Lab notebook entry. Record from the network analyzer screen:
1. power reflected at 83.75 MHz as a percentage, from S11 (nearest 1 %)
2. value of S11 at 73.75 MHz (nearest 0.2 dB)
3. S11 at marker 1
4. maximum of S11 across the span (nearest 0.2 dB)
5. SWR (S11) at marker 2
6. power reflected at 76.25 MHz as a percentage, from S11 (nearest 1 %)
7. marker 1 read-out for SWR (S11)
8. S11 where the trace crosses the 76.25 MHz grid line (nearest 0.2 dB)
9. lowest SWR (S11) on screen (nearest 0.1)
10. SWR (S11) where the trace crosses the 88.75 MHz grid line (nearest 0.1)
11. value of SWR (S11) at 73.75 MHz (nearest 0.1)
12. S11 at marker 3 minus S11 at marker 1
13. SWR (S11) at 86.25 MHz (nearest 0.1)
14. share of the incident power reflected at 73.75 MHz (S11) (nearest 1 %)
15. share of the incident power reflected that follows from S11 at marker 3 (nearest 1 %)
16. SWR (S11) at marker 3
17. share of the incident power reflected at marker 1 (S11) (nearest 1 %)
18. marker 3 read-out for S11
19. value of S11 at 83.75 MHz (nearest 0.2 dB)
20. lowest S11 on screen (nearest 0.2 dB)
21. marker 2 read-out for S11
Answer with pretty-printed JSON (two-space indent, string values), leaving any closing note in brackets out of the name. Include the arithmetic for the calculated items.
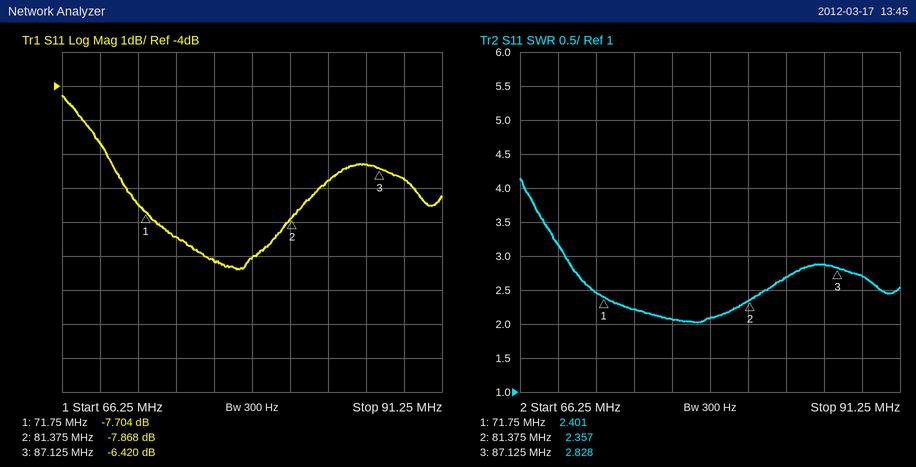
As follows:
{
  "power reflected at 83.75 MHz as a percentage, from S11": "10^(-6.8/10) ≈ 21 %",
  "value of S11 at 73.75 MHz": "-8.4 dB",
  "S11 at marker 1": "-7.704 dB",
  "maximum of S11 across the span": "-4.2 dB",
  "SWR (S11) at marker 2": "2.357",
  "power reflected at 76.25 MHz as a percentage, from S11": "10^(-9.2/10) ≈ 12 %",
  "marker 1 read-out for SWR": "2.401",
  "S11 where the trace crosses the 76.25 MHz grid line": "-9.2 dB",
  "lowest SWR (S11) on screen": "2.0",
  "SWR (S11) where the trace crosses the 88.75 MHz grid line": "2.7",
  "value of SWR (S11) at 73.75 MHz": "2.2",
  "S11 at marker 3 minus S11 at marker 1": "-6.42 − (-7.704) = 1.284 dB",
  "SWR (S11) at 86.25 MHz": "2.9",
  "share of the incident power reflected at 73.75 MHz (S11)": "10^(-8.4/10) ≈ 14 %",
  "share of the incident power reflected that follows from S11 at marker 3": "10^(-6.42/10) ≈ 23 %",
  "SWR (S11) at marker 3": "2.828",
  "share of the incident power reflected at marker 1 (S11)": "10^(-7.704/10) ≈ 17 %",
  "marker 3 read-out for S11": "-6.420 dB",
  "value of S11 at 83.75 MHz": "-6.8 dB",
  "lowest S11 on screen": "-9.4 dB",
  "marker 2 read-out for S11": "-7.868 dB"
}
